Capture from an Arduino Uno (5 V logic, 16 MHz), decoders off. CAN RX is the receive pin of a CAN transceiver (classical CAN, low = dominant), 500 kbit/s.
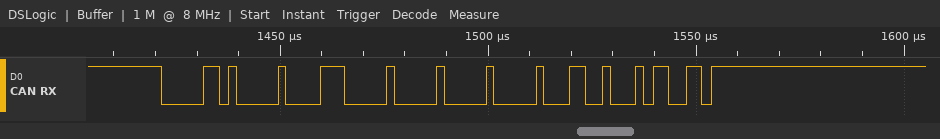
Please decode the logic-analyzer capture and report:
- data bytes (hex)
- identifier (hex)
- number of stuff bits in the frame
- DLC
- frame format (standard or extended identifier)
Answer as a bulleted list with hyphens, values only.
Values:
- 80 00 00
- 0x050
- 6
- 3
- standard
